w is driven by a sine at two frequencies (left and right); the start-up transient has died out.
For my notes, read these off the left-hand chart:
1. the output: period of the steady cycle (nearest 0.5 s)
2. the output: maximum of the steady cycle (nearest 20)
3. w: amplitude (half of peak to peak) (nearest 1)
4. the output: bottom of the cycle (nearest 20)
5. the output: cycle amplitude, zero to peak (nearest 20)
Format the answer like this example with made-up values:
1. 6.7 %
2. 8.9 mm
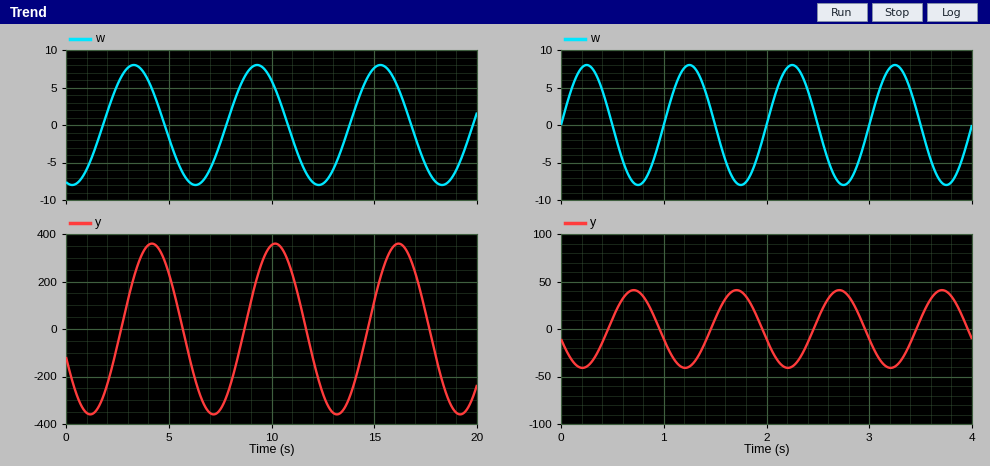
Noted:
1. 6.0 s
2. 360
3. 8
4. -360
5. 360
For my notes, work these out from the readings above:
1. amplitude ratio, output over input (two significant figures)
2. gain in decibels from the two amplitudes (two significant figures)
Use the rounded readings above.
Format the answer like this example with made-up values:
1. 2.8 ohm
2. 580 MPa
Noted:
1. 45
2. 33 dB
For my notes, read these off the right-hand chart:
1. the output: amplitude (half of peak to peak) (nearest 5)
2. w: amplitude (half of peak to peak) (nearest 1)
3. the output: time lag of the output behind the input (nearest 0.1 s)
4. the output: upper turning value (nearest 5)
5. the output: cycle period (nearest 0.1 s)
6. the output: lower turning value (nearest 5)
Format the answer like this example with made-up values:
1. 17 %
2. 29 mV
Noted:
1. 40
2. 8
3. 0.5 s
4. 40
5. 1.0 s
6. -40
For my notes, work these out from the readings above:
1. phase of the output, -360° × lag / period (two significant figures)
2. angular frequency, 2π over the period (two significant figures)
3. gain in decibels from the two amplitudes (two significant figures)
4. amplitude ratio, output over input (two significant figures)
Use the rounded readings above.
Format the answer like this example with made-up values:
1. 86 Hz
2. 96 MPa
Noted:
1. -180°
2. 6.3 rad/s
3. 14 dB
4. 5.0
